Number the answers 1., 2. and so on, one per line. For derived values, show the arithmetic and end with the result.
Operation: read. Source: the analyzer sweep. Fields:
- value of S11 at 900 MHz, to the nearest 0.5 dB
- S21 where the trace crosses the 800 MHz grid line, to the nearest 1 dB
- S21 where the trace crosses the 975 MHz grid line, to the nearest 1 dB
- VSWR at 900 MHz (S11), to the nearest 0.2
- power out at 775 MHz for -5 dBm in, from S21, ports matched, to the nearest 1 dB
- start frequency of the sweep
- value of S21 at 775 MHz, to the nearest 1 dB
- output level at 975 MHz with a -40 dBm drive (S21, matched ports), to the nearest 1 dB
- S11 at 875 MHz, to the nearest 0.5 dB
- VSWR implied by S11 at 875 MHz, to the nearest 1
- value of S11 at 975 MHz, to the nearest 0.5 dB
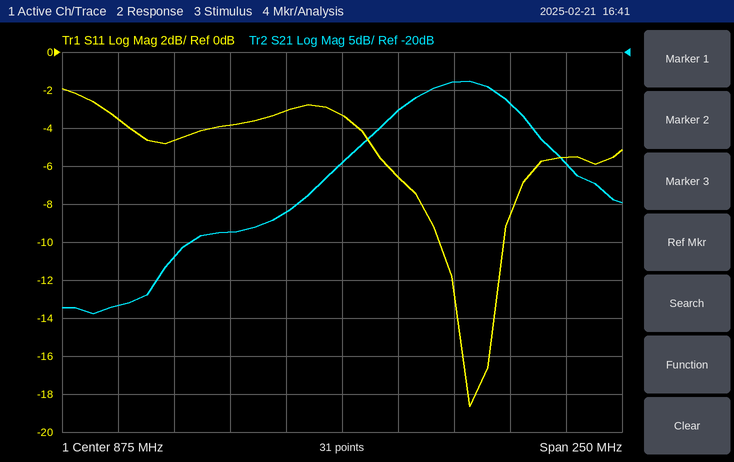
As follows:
1. -6.5 dB
2. -47 dB
3. -35 dB
4. |Γ| = 10^(-6.5/20) = 0.4732; VSWR = (1 + 0.4732)/(1 − 0.4732) ≈ 2.8
5. -5 dBm + (-53 dB) = -58 dBm
6. 750 MHz
7. -53 dB
8. -40 dBm + (-35 dB) = -75 dBm
9. -3.5 dB
10. |Γ| = 10^(-3.5/20) = 0.6683; VSWR = (1 + 0.6683)/(1 − 0.6683) ≈ 5
11. -5.5 dB
